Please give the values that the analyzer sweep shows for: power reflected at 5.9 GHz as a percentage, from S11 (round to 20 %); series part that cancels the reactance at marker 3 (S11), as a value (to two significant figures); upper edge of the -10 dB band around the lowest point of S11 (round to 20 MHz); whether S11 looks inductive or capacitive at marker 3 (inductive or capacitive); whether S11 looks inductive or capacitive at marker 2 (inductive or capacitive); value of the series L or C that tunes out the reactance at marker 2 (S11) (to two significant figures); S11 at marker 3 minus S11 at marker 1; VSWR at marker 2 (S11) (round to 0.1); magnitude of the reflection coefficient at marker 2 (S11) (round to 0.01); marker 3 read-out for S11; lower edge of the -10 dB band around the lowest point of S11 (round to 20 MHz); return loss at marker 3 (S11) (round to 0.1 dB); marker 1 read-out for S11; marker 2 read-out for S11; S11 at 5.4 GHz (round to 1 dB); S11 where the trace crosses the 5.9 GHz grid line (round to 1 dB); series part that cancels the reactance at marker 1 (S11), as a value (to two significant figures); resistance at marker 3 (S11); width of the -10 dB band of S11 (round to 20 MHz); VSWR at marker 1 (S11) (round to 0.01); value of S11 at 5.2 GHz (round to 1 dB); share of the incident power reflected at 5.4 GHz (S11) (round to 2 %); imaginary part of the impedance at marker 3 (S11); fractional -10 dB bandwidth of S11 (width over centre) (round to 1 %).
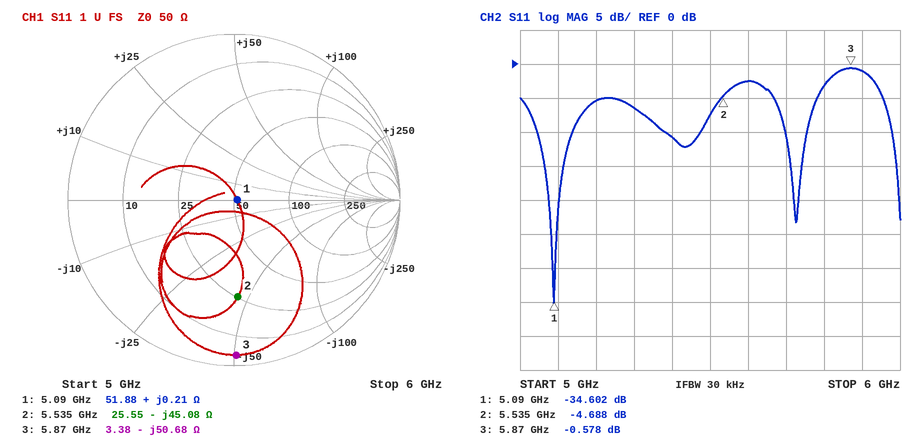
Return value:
80 %
1.4 nH
5.14 GHz
capacitive
capacitive
1.3 nH
34.024 dB
3.8
0.58
-0.578 dB
5.04 GHz
0.6 dB
-34.602 dB
-4.688 dB
-11 dB
-1 dB
150 pF
3.38 Ω
100 MHz
1.04
-5 dB
8 %
-50.68 Ω
2 %
